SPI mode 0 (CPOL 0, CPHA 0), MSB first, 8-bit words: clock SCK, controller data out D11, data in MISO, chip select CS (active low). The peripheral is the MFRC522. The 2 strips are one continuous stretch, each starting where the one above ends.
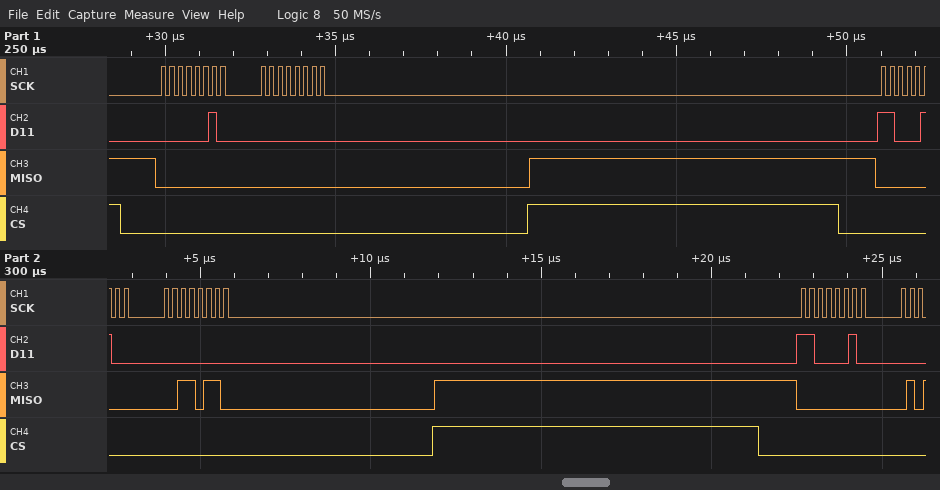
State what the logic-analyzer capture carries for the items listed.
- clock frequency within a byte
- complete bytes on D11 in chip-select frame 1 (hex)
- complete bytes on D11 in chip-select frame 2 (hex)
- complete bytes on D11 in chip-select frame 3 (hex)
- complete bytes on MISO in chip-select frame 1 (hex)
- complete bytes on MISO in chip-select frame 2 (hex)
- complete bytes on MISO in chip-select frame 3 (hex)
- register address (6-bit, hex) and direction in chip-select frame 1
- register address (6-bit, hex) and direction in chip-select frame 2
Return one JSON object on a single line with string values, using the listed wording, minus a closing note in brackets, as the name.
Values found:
{"clock frequency within a byte": "4 MHz", "complete bytes on D11 in chip-select frame 1": "02 00", "complete bytes on D11 in chip-select frame 2": "C4 00", "complete bytes on D11 in chip-select frame 3": "C2", "complete bytes on MISO in chip-select frame 1": "00 00", "complete bytes on MISO in chip-select frame 2": "00 36", "complete bytes on MISO in chip-select frame 3": "00", "register address (6-bit, hex) and direction in chip-select frame 1": "0x01 write", "register address (6-bit, hex) and direction in chip-select frame 2": "0x22 read"}
